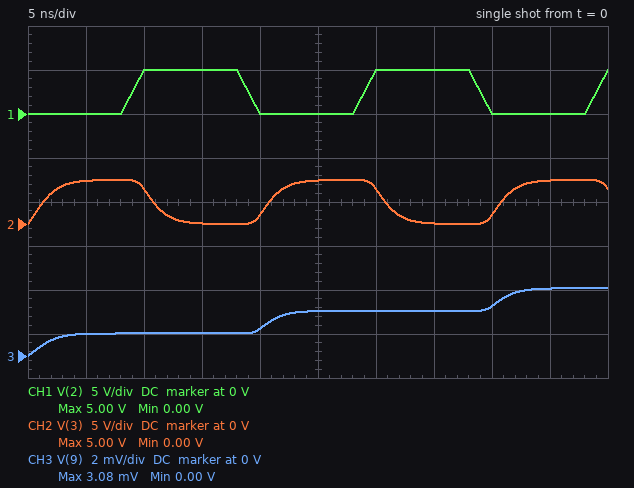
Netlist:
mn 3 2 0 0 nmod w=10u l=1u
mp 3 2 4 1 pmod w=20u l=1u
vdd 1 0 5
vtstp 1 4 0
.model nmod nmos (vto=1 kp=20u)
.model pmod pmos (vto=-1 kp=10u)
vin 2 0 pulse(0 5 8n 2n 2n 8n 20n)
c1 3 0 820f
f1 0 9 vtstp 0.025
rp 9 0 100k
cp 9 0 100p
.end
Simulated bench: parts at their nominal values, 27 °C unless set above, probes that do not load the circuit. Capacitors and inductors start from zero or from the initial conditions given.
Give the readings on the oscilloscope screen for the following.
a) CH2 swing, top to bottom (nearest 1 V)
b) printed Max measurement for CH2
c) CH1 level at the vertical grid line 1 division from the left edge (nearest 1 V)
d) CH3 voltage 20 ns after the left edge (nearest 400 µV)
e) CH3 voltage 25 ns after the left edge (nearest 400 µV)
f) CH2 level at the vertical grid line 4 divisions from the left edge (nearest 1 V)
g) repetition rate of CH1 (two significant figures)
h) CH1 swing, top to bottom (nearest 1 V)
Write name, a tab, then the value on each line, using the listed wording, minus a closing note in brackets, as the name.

CH2 swing, top to bottom	5 V
printed Max measurement for CH2	5.00 V
CH1 level at the vertical grid line 1 division from the left edge	0 V
CH3 voltage 20 ns after the left edge	1.2 mV
CH3 voltage 25 ns after the left edge	2.0 mV
CH2 level at the vertical grid line 4 divisions from the left edge	1 V
repetition rate of CH1	50 MHz
CH1 swing, top to bottom	5 V
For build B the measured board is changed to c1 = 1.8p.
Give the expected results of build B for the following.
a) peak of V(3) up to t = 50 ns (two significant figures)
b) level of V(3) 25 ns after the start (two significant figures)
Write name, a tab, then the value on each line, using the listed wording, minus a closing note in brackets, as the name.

peak of V(3) up to t = 50 ns	4.8 V
level of V(3) 25 ns after the start	4.1 V
